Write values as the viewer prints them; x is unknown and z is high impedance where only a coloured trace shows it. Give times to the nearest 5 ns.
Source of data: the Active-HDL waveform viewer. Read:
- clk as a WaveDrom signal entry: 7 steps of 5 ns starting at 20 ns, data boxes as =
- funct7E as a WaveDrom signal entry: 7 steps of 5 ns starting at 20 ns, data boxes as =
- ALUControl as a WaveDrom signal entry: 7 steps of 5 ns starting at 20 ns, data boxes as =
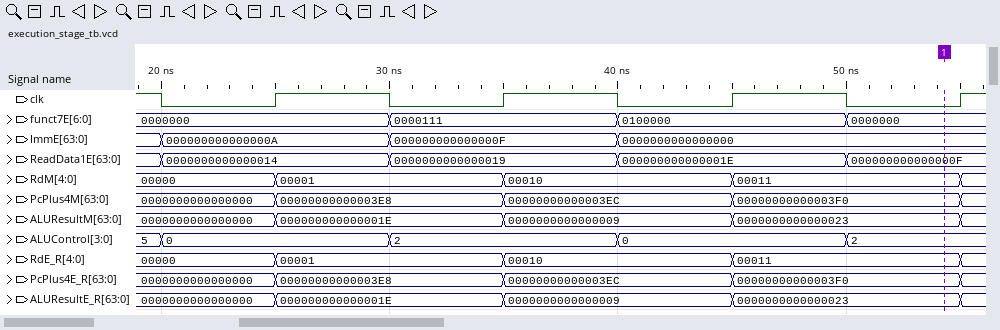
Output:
{name: 'clk', wave: '0101010'}
{name: 'funct7E', wave: '=.=.=.=', data: '0000000 0000111 0100000 0000000'}
{name: 'ALUControl', wave: '=.=.=.=', data: '0 2 0 2'}
